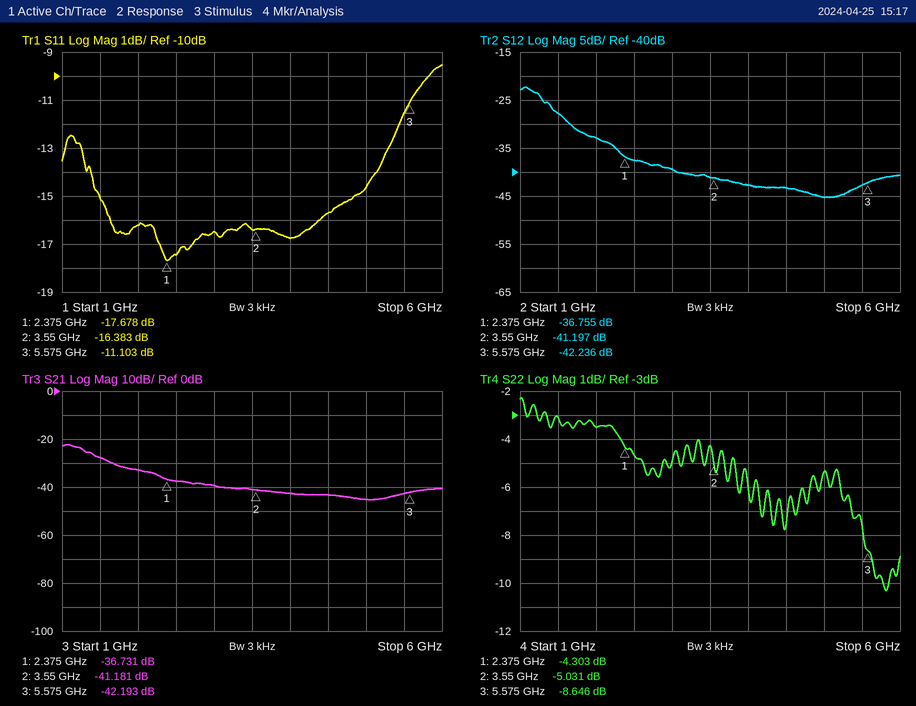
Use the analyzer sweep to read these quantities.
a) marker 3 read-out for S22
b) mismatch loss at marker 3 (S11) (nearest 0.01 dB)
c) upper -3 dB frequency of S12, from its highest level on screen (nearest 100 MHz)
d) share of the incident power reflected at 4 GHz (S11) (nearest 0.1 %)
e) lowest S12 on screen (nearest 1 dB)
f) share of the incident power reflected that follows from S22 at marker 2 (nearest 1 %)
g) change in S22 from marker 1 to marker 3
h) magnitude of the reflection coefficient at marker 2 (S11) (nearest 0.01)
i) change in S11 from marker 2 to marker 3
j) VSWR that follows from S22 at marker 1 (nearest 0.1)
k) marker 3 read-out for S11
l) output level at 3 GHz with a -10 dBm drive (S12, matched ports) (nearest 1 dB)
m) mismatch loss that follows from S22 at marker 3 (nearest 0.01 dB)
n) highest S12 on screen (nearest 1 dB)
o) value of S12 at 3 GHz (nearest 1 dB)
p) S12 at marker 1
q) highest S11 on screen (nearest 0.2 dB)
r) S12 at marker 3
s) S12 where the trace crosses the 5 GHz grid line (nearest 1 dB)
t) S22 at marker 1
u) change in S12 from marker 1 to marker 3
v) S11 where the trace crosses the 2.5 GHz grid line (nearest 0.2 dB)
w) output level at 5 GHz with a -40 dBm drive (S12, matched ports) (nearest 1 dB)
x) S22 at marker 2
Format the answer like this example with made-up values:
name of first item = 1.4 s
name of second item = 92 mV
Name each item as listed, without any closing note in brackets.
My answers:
marker 3 read-out for S22 = -8.646 dB
mismatch loss at marker 3 (S11) = 0.35 dB
upper -3 dB frequency of S12, from its highest level on screen = 1.3 GHz
share of the incident power reflected at 4 GHz (S11) = 2.1 %
lowest S12 on screen = -45 dB
share of the incident power reflected that follows from S22 at marker 2 = 31 %
change in S22 from marker 1 to marker 3 = -4.343 dB
magnitude of the reflection coefficient at marker 2 (S11) = 0.15
change in S11 from marker 2 to marker 3 = 5.280 dB
VSWR that follows from S22 at marker 1 = 4.1
marker 3 read-out for S11 = -11.103 dB
output level at 3 GHz with a -10 dBm drive (S12, matched ports) = -49 dBm
mismatch loss that follows from S22 at marker 3 = 0.64 dB
highest S12 on screen = -22 dB
value of S12 at 3 GHz = -39 dB
S12 at marker 1 = -36.755 dB
highest S11 on screen = -9.6 dB
S12 at marker 3 = -42.236 dB
S12 where the trace crosses the 5 GHz grid line = -45 dB
S22 at marker 1 = -4.303 dB
change in S12 from marker 1 to marker 3 = -5.481 dB
S11 where the trace crosses the 2.5 GHz grid line = -17.4 dB
output level at 5 GHz with a -40 dBm drive (S12, matched ports) = -85 dBm
S22 at marker 2 = -5.031 dB
